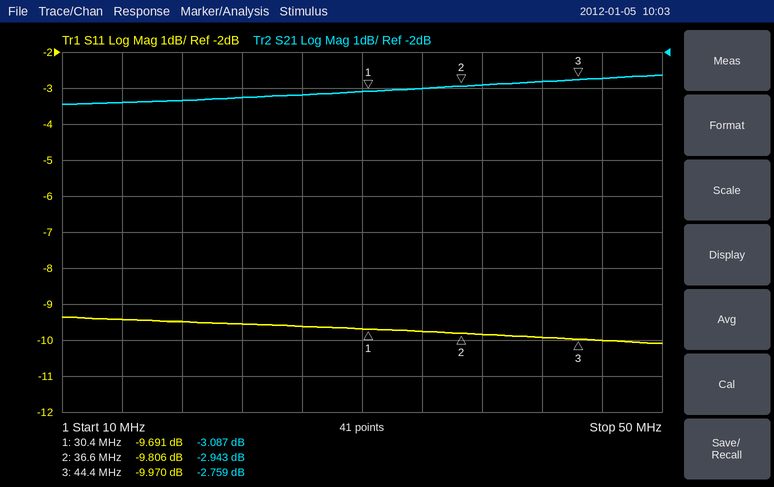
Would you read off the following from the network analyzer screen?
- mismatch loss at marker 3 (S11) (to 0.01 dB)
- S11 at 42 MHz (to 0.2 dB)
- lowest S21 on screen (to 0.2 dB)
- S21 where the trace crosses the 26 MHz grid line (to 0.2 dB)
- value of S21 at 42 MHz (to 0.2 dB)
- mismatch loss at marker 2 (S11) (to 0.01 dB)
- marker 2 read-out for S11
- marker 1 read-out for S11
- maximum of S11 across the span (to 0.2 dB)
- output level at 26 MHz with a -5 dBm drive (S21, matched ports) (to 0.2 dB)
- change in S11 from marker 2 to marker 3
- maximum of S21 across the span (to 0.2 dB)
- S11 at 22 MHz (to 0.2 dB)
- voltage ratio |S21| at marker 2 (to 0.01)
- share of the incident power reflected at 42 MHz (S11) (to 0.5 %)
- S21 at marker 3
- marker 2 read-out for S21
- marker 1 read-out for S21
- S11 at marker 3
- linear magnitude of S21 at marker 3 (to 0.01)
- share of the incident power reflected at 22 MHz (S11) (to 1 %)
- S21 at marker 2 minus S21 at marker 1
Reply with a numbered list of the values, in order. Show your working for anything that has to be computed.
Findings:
1. −10 log10(1 − 10^(-9.97/10)) ≈ 0.46 dB
2. -10.0 dB
3. -3.4 dB
4. -3.2 dB
5. -2.8 dB
6. −10 log10(1 − 10^(-9.806/10)) ≈ 0.48 dB
7. -9.806 dB
8. -9.691 dB
9. -9.4 dB
10. -5 dBm + (-3.2 dB) = -8.2 dBm
11. -9.97 − (-9.806) = -0.164 dB
12. -2.6 dB
13. -9.6 dB
14. 10^(-2.943/20) ≈ 0.71
15. 10^(-10/10) ≈ 10.0 %
16. -2.759 dB
17. -2.943 dB
18. -3.087 dB
19. -9.970 dB
20. 10^(-2.759/20) ≈ 0.73
21. 10^(-9.6/10) ≈ 11 %
22. -2.943 − (-3.087) = 0.144 dB
